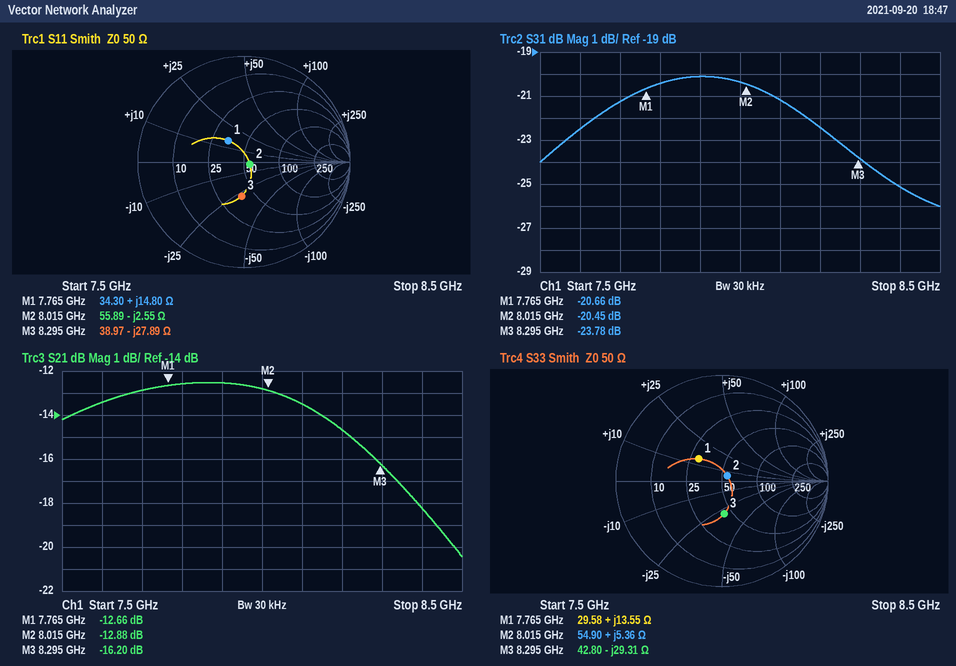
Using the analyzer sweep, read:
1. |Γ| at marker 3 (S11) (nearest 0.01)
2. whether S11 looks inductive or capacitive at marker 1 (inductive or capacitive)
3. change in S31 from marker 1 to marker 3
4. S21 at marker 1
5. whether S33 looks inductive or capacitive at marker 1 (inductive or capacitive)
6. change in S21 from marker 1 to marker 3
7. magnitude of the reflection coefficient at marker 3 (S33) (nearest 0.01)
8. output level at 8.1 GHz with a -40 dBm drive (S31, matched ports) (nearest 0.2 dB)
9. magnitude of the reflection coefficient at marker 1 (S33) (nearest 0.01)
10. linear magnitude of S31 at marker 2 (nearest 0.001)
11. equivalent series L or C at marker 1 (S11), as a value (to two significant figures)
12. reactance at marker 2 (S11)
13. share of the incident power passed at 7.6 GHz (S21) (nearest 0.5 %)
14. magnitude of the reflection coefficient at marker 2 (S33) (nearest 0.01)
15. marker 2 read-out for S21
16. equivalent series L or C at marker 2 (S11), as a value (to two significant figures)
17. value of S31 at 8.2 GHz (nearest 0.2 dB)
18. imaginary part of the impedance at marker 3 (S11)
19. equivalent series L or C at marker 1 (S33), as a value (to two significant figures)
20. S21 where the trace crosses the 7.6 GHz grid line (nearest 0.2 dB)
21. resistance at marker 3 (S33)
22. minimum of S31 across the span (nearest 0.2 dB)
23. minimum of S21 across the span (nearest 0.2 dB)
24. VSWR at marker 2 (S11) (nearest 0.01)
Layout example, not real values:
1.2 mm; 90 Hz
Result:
0.32; inductive; -3.12 dB; -12.66 dB; inductive; -3.54 dB; 0.31; -61.2 dBm; 0.30; 0.095; 300 pH; -2.55 Ω; 4.5 %; 0.07; -12.88 dB; 7.8 pF; -22.4 dB; -27.89 Ω; 280 pH; -13.4 dB; 42.80 Ω; -26.0 dB; -20.4 dB; 1.13
